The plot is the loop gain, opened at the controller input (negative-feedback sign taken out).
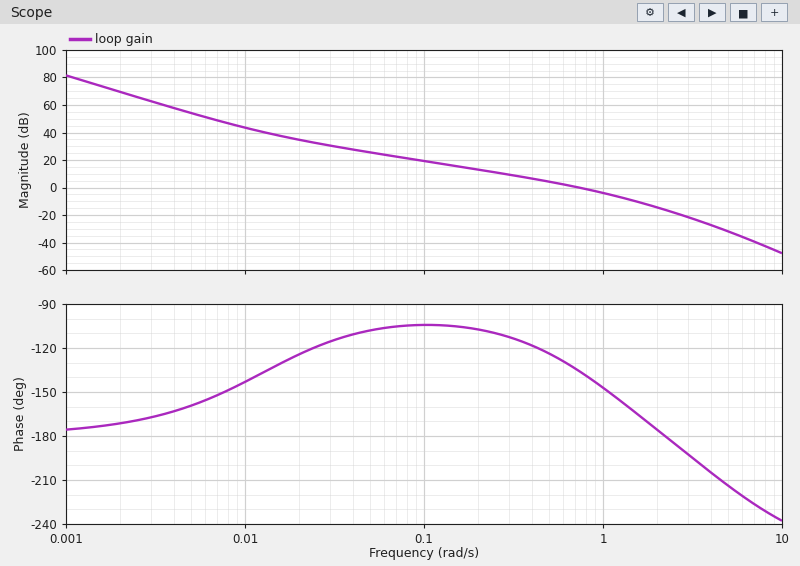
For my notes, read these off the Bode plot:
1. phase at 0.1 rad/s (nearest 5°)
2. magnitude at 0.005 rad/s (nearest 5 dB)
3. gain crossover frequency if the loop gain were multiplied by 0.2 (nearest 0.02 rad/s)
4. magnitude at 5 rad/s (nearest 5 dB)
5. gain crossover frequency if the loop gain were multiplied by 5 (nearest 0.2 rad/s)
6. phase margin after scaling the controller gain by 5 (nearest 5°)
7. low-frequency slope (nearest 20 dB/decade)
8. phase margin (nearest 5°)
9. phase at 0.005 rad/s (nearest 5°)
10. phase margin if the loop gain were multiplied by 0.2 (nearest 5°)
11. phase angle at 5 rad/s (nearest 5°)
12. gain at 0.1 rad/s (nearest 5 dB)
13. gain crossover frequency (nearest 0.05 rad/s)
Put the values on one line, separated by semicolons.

-105°; 55 dB; 0.18 rad/s; -30 dB; 2.0 rad/s; 5°; -40 dB/decade; 45°; -160°; 75°; -215°; 20 dB; 0.75 rad/s
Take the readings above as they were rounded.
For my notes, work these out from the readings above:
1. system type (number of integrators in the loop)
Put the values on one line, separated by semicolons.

2
